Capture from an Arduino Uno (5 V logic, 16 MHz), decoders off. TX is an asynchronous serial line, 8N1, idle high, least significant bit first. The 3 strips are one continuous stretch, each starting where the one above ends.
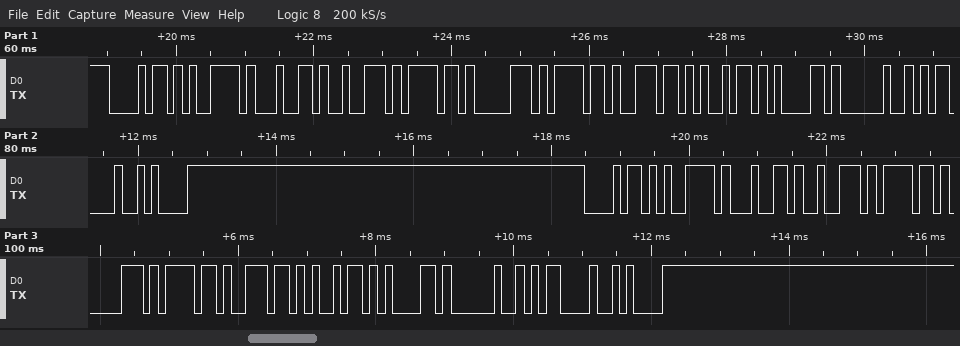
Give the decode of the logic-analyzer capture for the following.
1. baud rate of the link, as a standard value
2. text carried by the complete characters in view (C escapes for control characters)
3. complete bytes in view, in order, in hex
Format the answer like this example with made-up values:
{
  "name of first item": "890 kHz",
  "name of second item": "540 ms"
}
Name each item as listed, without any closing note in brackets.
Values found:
{
  "baud rate of the link, as a standard value": "9600 baud",
  "text carried by the complete characters in view": "\"hydroponia \\r\\nhydroponia \\r\\n\"",
  "complete bytes in view, in order, in hex": "68 79 64 72 6F 70 6F 6E 69 61 20 0D 0A 68 79 64 72 6F 70 6F 6E 69 61 20 0D 0A"
}
